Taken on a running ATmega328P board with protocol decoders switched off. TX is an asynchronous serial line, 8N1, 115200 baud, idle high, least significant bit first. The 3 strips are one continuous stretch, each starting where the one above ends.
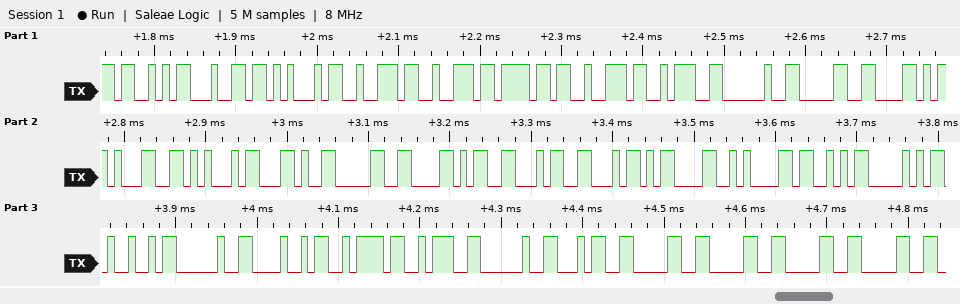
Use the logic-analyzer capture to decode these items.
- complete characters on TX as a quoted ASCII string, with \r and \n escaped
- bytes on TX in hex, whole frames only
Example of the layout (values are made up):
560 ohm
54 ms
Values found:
"SdError: 0X1E,0XFF\r\nSPI Hz: 40000"
53 64 45 72 72 6F 72 3A 20 30 58 31 45 2C 30 58 46 46 0D 0A 53 50 49 20 48 7A 3A 20 34 30 30 30 30
